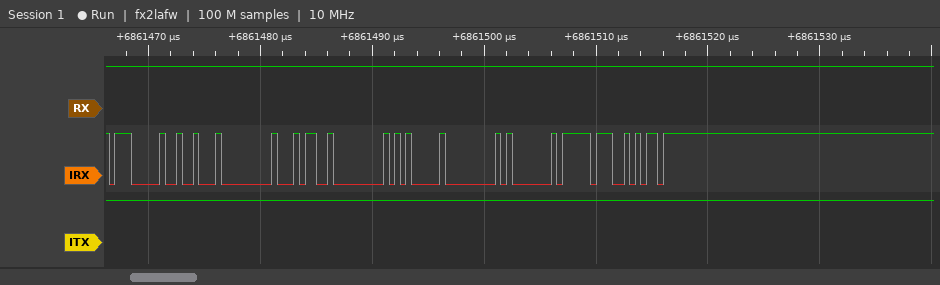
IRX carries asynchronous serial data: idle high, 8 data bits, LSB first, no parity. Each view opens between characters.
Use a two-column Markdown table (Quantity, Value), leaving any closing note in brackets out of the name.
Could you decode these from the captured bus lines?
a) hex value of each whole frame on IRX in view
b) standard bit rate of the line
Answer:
| Quantity | Value |
|---|---|
| hex value of each whole frame on IRX in view | 07, 12, 00, 34, 00, 05, 00, 01, DF, 6A |
| standard bit rate of the line | 2000000 baud |
